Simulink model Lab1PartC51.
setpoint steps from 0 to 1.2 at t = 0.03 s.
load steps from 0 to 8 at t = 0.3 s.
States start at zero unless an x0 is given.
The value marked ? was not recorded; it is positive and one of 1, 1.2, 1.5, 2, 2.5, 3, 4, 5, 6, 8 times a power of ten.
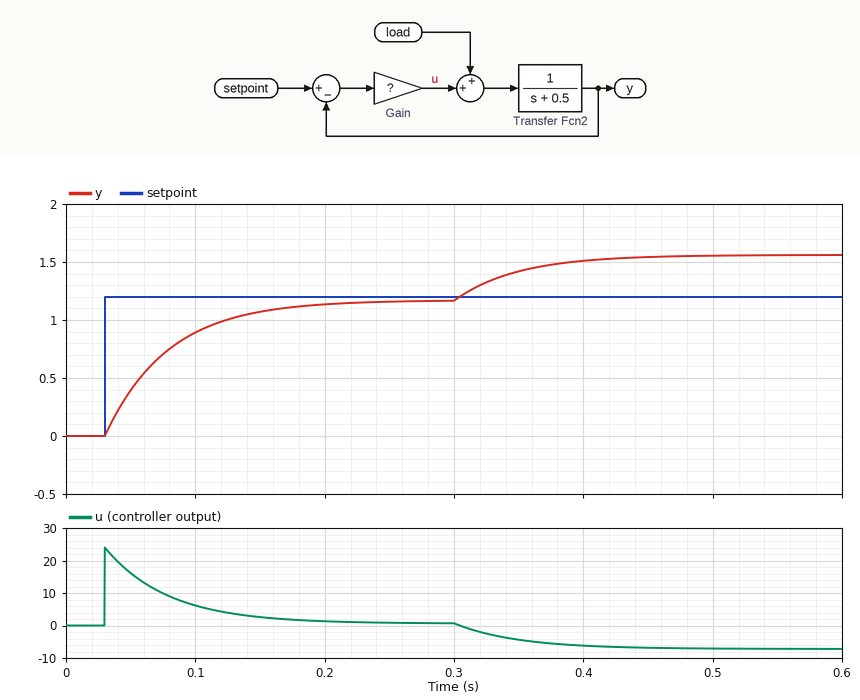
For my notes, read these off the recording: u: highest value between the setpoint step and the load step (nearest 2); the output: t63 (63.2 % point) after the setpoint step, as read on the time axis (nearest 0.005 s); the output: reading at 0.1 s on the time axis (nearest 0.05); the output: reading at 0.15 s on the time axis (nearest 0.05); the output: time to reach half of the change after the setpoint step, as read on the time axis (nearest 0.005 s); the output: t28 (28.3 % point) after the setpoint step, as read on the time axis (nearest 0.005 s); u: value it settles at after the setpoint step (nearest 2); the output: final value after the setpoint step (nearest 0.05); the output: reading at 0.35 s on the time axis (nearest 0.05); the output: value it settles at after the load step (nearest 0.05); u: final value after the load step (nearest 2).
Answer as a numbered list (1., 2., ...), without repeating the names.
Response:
1. 24
2. 0.080 s
3. 0.90
4. 1.05
5. 0.065 s
6. 0.045 s
7. 0
8. 1.15
9. 1.40
10. 1.55
11. -8
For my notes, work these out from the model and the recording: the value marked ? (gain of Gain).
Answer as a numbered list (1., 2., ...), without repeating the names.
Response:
1. 20
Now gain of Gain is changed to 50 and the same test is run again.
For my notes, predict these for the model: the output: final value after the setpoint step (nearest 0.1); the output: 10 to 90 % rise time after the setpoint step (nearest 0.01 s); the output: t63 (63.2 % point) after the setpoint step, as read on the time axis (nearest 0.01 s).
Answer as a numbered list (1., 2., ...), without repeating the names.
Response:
1. 1.2
2. 0.04 s
3. 0.05 s
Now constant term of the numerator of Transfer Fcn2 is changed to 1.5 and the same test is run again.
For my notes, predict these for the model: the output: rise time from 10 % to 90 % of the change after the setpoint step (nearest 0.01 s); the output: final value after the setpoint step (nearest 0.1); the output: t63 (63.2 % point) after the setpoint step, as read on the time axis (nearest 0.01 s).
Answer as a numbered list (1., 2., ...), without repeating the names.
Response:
1. 0.07 s
2. 1.2
3. 0.06 s
